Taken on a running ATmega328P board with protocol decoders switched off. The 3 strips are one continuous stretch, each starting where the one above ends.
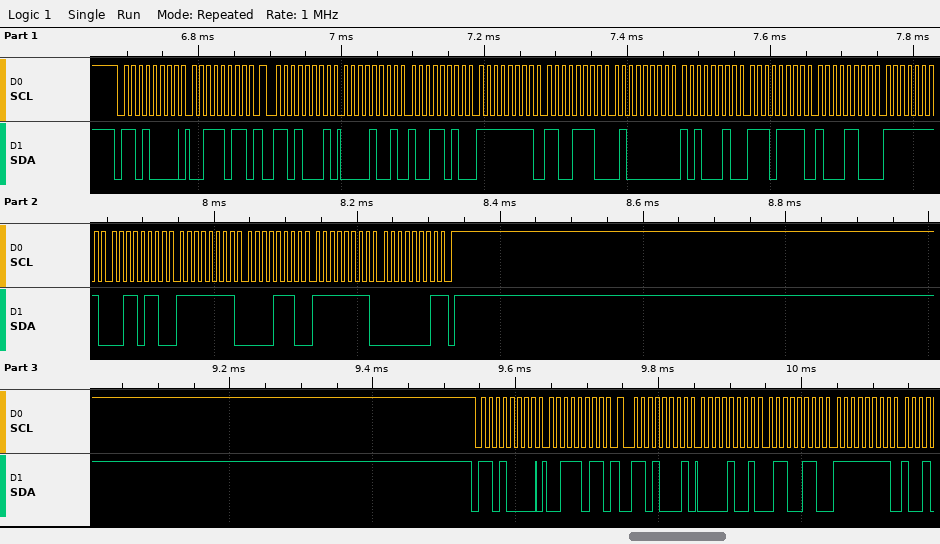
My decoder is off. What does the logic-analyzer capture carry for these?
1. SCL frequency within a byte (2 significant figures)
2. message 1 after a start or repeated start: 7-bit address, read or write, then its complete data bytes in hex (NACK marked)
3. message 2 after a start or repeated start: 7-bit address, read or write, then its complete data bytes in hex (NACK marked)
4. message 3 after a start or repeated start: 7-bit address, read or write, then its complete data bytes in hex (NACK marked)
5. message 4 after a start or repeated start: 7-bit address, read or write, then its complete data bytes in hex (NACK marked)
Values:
100 kHz
0x68 write: 3B
0x68 read: 09 9A FF CE 40 A2 EF 8C FF 36 FF 0E FF 01 NACK
0x68 write: 3B
0x68 read: 09 66 FF
